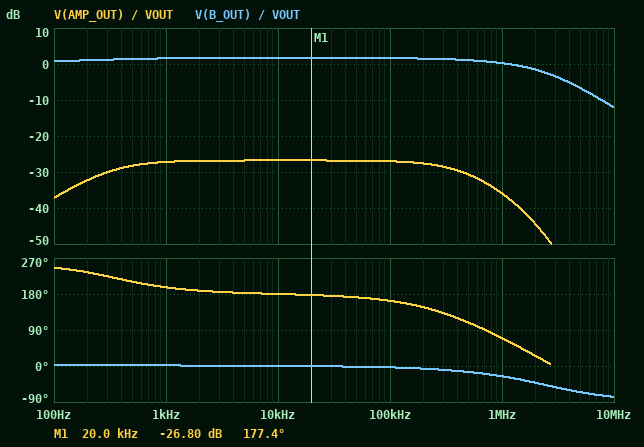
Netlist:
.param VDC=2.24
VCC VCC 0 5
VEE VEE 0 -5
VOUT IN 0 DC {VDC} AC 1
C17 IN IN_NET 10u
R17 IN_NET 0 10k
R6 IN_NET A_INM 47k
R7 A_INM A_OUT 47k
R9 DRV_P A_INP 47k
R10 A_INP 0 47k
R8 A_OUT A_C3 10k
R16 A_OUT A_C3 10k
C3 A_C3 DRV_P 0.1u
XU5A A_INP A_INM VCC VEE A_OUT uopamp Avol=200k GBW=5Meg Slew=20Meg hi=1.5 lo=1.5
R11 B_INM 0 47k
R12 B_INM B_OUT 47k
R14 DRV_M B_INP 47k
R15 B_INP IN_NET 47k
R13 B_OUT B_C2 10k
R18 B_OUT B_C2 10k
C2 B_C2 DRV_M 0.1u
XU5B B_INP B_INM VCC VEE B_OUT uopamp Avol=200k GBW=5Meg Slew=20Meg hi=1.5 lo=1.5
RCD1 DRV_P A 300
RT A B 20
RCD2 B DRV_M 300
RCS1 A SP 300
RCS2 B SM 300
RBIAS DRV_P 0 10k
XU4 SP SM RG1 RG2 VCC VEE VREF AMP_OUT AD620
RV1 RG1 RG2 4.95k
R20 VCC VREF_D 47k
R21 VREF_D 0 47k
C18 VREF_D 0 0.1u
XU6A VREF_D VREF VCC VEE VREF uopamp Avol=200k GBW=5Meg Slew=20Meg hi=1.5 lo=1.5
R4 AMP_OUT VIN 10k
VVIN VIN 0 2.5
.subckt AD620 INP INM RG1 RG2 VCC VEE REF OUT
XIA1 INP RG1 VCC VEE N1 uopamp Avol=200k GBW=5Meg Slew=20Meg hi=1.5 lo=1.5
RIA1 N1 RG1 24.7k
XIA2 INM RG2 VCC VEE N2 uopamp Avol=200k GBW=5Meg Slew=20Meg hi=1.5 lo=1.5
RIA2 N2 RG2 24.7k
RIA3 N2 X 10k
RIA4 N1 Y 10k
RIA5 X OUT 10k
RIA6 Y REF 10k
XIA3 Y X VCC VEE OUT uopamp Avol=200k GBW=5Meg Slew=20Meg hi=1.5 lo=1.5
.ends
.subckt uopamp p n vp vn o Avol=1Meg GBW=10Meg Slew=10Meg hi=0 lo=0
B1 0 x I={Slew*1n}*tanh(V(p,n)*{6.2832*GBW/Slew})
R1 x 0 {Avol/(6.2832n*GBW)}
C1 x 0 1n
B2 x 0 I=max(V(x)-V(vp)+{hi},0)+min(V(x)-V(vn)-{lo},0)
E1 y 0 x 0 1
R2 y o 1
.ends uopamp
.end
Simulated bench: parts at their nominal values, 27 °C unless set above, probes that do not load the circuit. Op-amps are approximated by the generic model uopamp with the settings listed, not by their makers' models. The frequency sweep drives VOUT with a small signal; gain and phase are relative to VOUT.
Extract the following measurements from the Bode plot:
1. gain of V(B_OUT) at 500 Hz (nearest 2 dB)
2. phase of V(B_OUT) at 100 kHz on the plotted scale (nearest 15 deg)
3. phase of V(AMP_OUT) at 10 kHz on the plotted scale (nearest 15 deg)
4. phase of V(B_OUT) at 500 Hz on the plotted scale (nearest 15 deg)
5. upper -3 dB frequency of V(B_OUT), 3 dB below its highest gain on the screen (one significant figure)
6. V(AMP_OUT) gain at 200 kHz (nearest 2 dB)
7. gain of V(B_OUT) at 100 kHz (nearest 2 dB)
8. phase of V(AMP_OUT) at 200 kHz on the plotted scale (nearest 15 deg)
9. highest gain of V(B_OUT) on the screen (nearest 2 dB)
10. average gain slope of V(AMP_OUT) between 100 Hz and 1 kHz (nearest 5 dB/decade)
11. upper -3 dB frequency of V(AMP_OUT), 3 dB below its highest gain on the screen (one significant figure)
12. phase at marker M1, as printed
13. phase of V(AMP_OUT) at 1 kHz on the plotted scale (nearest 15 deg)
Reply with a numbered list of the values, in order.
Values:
1. 2 dB
2. 0 deg
3. 180 deg
4. 0 deg
5. 2 MHz
6. -28 dB
7. 2 dB
8. 150 deg
9. 2 dB
10. 10 dB/decade
11. 400 kHz
12. 177.4 deg
13. 195 deg
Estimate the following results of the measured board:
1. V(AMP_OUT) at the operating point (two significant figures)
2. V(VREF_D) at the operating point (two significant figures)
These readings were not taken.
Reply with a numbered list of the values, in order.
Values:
1. 2.5 V
2. 2.5 V
